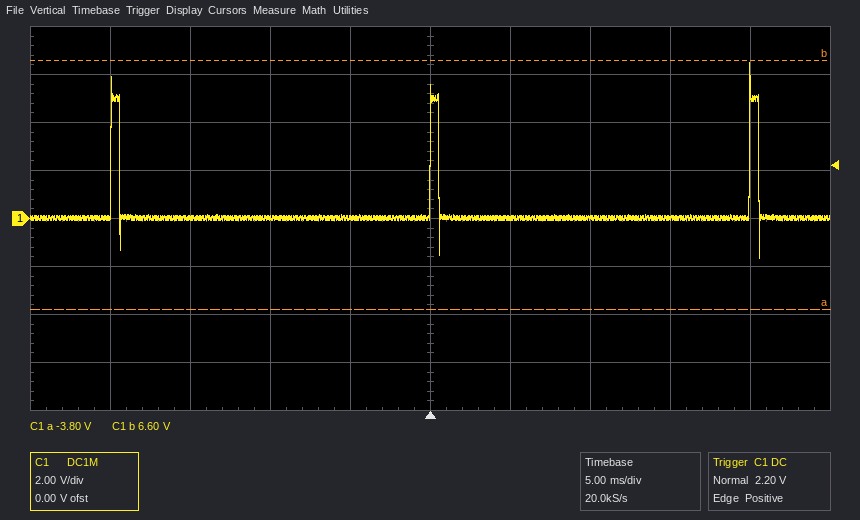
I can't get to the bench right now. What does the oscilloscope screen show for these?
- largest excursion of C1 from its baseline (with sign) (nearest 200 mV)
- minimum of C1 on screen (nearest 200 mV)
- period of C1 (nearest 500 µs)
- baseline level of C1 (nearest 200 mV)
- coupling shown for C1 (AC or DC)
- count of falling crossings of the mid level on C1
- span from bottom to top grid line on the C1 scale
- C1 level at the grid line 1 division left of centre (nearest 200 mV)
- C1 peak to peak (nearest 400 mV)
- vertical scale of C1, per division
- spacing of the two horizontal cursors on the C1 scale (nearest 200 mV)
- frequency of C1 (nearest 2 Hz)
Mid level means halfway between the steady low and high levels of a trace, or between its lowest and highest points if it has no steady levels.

+6.4 V
-1.6 V
20.0 ms
0.0 V
DC
3
16 V
0.0 V
8.0 V
2 V
10.4 V
50 Hz
